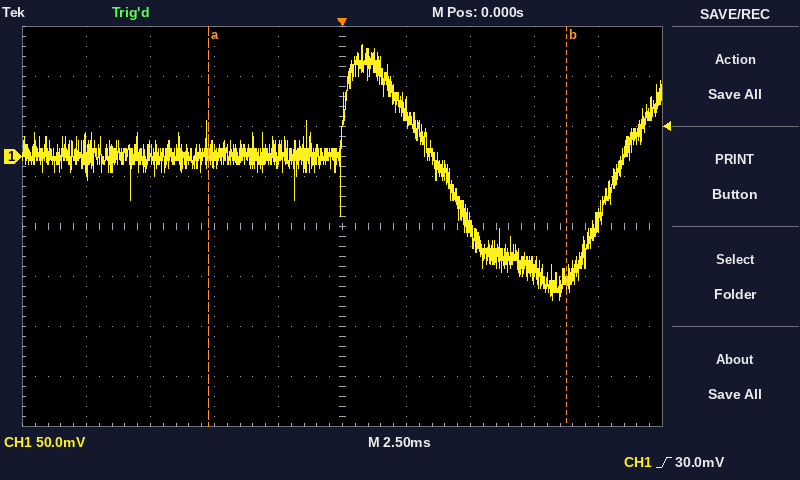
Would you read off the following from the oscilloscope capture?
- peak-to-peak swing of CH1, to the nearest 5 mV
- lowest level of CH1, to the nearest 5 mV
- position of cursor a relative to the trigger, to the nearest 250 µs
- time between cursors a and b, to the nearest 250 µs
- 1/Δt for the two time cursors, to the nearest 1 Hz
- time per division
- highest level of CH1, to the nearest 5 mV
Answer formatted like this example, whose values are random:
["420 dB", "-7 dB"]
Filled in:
["255 mV", "-145 mV", "-5.25 ms", "14.00 ms", "71 Hz", "2.5 ms", "110 mV"]
